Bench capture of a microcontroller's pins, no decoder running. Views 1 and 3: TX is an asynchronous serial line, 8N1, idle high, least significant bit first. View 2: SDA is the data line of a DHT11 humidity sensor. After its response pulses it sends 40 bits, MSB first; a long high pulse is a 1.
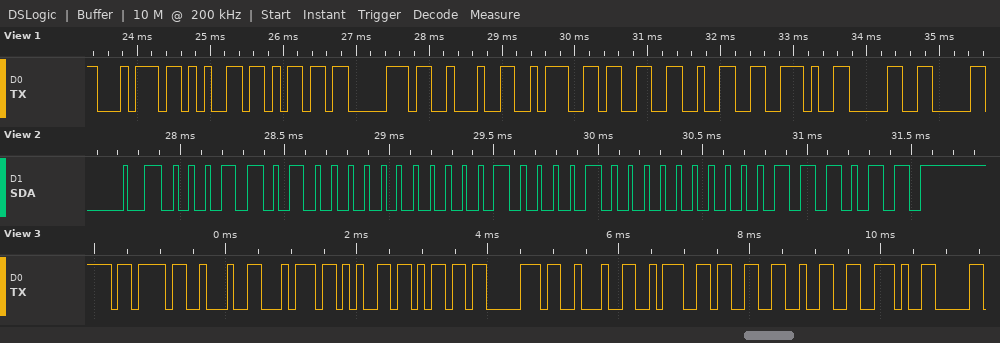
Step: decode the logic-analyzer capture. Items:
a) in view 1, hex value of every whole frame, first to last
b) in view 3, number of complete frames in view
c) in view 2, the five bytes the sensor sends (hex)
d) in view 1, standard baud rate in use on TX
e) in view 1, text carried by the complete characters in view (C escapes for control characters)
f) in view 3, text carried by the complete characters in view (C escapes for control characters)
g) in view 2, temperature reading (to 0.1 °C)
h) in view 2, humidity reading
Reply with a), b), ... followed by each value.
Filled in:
a) 74 65 6D 70 22 3A 33 32 2E 30
b) 11
c) 1A 00 21 00 3B
d) 9600 baud
e) "temp\":32.0"
f) "{\"temp\":32."
g) 33.0 °C
h) 26 %
